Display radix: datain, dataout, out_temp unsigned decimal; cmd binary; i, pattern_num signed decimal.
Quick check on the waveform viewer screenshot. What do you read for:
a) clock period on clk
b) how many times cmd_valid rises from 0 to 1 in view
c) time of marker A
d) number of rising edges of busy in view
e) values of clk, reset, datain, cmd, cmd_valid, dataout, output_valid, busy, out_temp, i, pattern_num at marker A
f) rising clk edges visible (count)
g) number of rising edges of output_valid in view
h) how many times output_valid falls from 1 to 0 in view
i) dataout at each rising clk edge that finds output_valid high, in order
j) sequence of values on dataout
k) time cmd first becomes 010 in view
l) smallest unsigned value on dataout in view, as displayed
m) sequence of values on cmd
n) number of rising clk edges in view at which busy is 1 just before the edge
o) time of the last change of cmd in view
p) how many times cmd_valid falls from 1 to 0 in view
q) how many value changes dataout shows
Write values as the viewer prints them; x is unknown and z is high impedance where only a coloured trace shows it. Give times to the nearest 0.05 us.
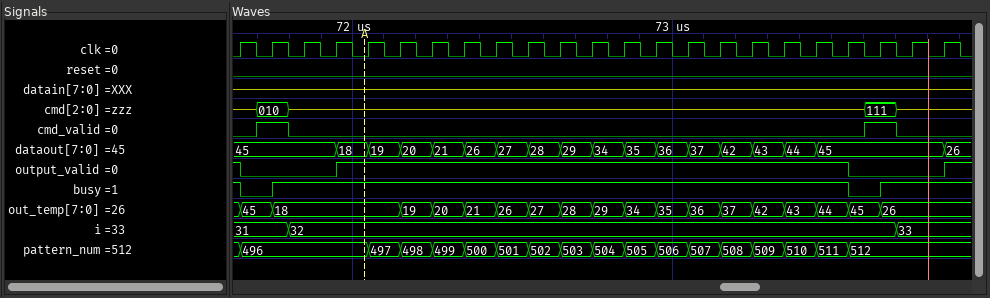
0.1 us
2
72.05 us
2
clk=0, reset=0, datain=z, cmd=z, cmd_valid=0, dataout=18, output_valid=1, busy=1, out_temp=18, i=32, pattern_num=496
23
2
2
45, 18, 19, 20, 21, 26, 27, 28, 29, 34, 35, 36, 37, 42, 43, 44, 45
45, 18, 19, 20, 21, 26, 27, 28, 29, 34, 35, 36, 37, 42, 43, 44, 45, 26
71.7 us
18
z, 010, z, 111, z
21
73.7 us
2
17
